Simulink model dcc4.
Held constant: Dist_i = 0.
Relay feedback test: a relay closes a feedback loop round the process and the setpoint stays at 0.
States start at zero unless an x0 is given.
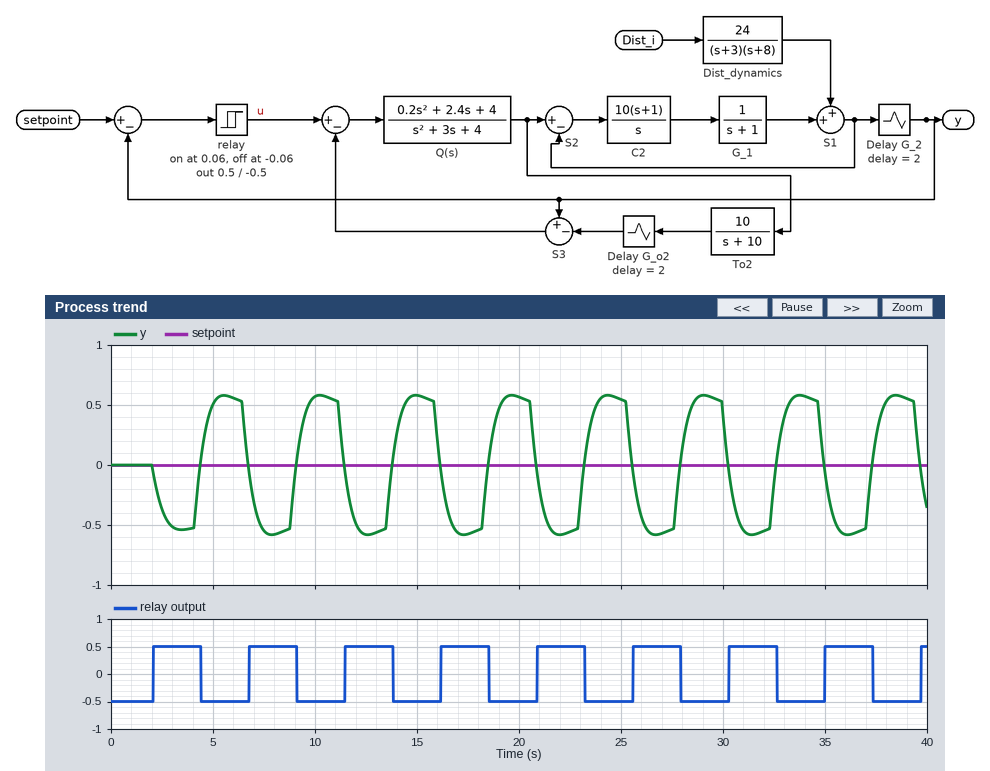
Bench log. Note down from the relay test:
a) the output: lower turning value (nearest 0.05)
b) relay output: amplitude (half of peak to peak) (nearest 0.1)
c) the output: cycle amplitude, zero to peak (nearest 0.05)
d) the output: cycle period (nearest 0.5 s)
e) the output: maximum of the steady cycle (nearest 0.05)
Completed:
-0.60
0.5
0.60
4.5 s
0.60
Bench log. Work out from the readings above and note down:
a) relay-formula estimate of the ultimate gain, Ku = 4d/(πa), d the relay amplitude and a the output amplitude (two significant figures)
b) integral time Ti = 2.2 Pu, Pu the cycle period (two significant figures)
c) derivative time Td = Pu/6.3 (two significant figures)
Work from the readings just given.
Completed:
1.1
9.9 s
0.71 s
